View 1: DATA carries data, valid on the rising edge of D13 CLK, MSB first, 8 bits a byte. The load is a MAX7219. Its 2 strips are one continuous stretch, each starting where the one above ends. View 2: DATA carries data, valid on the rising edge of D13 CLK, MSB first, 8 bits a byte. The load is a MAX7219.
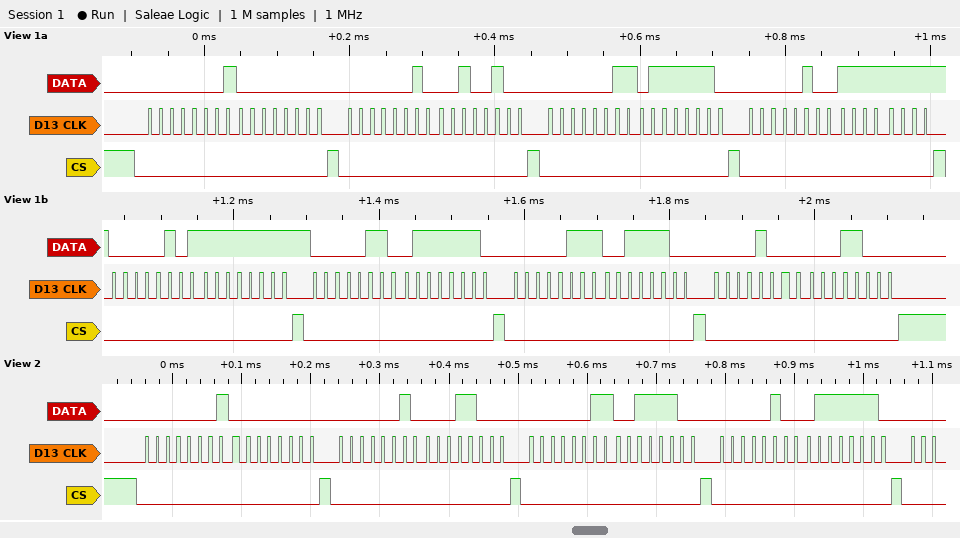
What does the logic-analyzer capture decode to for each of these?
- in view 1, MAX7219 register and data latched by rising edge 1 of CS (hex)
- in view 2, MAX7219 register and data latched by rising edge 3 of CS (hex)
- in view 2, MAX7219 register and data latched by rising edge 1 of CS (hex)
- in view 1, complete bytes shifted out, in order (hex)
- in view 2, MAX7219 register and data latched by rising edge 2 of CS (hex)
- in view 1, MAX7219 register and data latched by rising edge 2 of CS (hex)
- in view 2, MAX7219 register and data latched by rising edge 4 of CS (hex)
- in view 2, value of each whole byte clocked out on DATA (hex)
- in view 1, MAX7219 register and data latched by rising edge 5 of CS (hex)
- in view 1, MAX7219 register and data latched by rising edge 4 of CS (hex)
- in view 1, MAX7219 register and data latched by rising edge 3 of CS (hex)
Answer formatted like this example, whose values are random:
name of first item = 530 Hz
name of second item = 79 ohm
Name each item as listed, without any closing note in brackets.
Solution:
in view 1, MAX7219 register and data latched by rising edge 1 of CS = register 0x1, data 0x00
in view 2, MAX7219 register and data latched by rising edge 3 of CS = register 0x3, data 0x3C
in view 2, MAX7219 register and data latched by rising edge 1 of CS = register 0x1, data 0x00
in view 1, complete bytes shifted out, in order = 0x01 0x00 0x02 0x24 0x03 0x7E 0x04 0xFF 0x05 0xFF 0x06 0x7E 0x07 0x3C 0x08 0x18
in view 2, MAX7219 register and data latched by rising edge 2 of CS = register 0x2, data 0x18
in view 1, MAX7219 register and data latched by rising edge 2 of CS = register 0x2, data 0x24
in view 2, MAX7219 register and data latched by rising edge 4 of CS = register 0x4, data 0x7E
in view 2, value of each whole byte clocked out on DATA = 0x01 0x00 0x02 0x18 0x03 0x3C 0x04 0x7E
in view 1, MAX7219 register and data latched by rising edge 5 of CS = register 0x5, data 0xFF
in view 1, MAX7219 register and data latched by rising edge 4 of CS = register 0x4, data 0xFF
in view 1, MAX7219 register and data latched by rising edge 3 of CS = register 0x3, data 0x7E
